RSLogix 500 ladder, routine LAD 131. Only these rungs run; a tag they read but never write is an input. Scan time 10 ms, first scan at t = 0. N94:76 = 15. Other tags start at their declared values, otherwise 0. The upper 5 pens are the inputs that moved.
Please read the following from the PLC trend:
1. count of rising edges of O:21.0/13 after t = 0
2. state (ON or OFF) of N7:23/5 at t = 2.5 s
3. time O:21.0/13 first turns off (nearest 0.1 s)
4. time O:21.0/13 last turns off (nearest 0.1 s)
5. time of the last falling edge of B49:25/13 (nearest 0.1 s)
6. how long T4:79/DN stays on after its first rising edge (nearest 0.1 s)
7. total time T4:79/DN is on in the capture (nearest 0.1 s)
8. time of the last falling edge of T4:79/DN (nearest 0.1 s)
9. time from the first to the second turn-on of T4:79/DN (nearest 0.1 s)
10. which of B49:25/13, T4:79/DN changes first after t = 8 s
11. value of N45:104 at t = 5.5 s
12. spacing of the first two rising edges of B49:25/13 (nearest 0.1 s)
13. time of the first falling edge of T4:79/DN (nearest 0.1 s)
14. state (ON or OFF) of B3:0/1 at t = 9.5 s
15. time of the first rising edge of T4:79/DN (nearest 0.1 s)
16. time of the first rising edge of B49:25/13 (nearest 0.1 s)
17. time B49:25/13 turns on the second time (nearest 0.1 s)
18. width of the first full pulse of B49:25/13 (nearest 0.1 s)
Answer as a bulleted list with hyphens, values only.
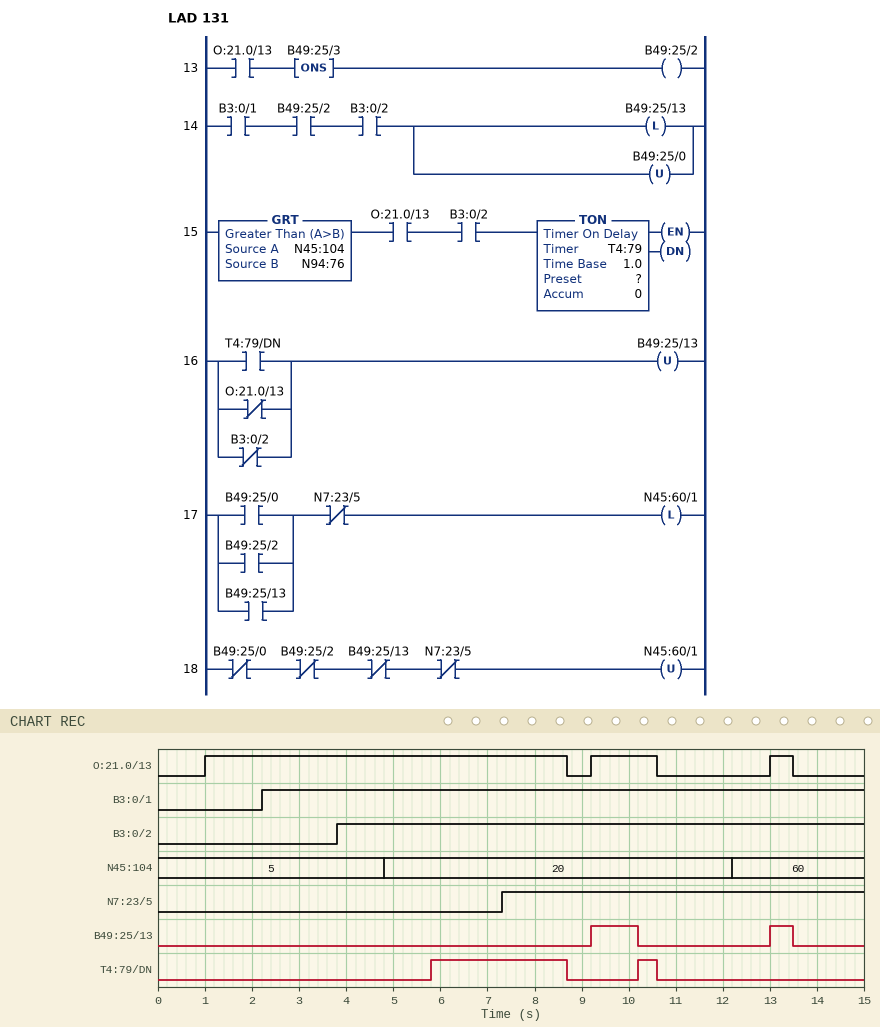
- 3
- OFF
- 8.7 s
- 13.5 s
- 13.5 s
- 2.9 s
- 3.3 s
- 10.6 s
- 4.4 s
- T4:79/DN
- 20
- 3.8 s
- 8.7 s
- ON
- 5.8 s
- 9.2 s
- 13.0 s
- 1.0 s
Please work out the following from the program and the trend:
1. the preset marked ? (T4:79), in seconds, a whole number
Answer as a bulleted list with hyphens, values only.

- 1 s
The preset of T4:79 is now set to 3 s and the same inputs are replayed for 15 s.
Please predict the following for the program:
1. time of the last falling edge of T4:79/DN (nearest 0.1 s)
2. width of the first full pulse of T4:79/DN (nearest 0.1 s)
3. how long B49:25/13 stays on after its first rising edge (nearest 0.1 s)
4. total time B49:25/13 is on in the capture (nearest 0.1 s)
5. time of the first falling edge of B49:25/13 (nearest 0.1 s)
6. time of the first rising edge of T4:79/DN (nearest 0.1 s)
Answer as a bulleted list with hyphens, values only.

- 8.7 s
- 0.9 s
- 1.4 s
- 1.9 s
- 10.6 s
- 7.8 s
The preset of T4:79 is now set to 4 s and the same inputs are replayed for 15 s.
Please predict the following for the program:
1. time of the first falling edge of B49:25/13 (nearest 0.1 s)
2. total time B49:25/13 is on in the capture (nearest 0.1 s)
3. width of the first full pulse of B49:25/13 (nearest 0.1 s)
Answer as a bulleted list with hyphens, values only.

- 10.6 s
- 1.9 s
- 1.4 s
